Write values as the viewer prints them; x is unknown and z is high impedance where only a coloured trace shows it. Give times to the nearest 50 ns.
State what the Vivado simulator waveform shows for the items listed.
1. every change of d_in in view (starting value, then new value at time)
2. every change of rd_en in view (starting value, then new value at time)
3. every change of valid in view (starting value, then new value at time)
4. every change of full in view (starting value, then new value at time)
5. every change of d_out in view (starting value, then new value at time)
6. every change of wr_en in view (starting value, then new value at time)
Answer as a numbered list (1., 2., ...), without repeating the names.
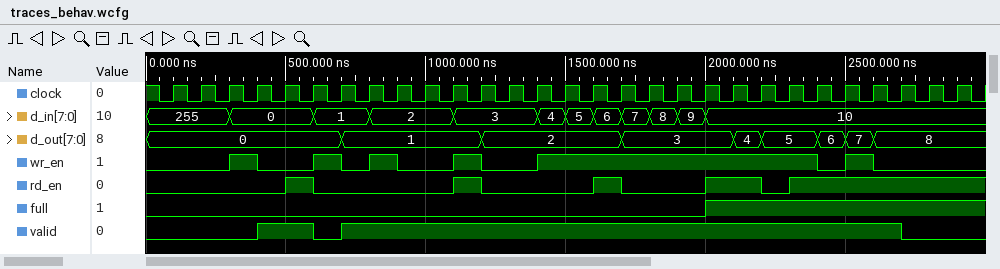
1. 255, 0 at 300 ns, 1 at 600 ns, 2 at 800 ns, 3 at 1100 ns, 4 at 1400 ns, 5 at 1500 ns, 6 at 1600 ns, 7 at 1700 ns, 8 at 1800 ns, 9 at 1900 ns, 10 at 2000 ns
2. 0, 1 at 500 ns, 0 at 600 ns, 1 at 1100 ns, 0 at 1200 ns, 1 at 1600 ns, 0 at 1700 ns, 1 at 2000 ns, 0 at 2200 ns, 1 at 2300 ns
3. 0, 1 at 400 ns, 0 at 600 ns, 1 at 700 ns, 0 at 2700 ns
4. 0, 1 at 2000 ns
5. 0, 1 at 700 ns, 2 at 1200 ns, 3 at 1700 ns, 4 at 2100 ns, 5 at 2200 ns, 6 at 2400 ns, 7 at 2500 ns, 8 at 2600 ns
6. 0, 1 at 300 ns, 0 at 400 ns, 1 at 600 ns, 0 at 700 ns, 1 at 800 ns, 0 at 900 ns, 1 at 1100 ns, 0 at 1200 ns, 1 at 1400 ns, 0 at 2400 ns, 1 at 2500 ns, 0 at 2600 ns
